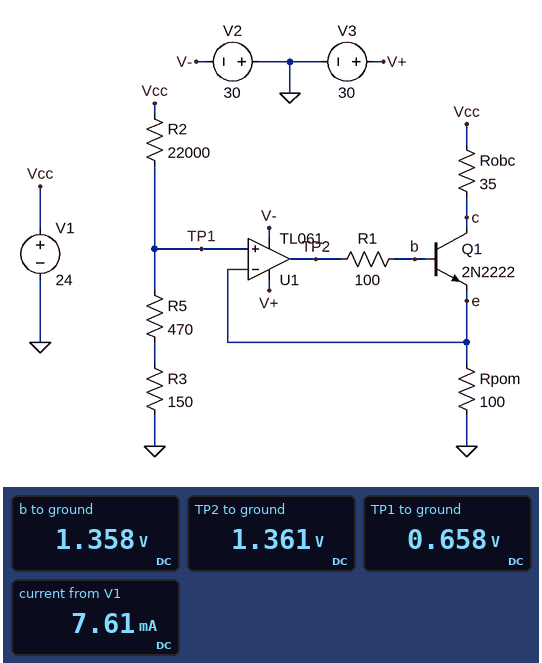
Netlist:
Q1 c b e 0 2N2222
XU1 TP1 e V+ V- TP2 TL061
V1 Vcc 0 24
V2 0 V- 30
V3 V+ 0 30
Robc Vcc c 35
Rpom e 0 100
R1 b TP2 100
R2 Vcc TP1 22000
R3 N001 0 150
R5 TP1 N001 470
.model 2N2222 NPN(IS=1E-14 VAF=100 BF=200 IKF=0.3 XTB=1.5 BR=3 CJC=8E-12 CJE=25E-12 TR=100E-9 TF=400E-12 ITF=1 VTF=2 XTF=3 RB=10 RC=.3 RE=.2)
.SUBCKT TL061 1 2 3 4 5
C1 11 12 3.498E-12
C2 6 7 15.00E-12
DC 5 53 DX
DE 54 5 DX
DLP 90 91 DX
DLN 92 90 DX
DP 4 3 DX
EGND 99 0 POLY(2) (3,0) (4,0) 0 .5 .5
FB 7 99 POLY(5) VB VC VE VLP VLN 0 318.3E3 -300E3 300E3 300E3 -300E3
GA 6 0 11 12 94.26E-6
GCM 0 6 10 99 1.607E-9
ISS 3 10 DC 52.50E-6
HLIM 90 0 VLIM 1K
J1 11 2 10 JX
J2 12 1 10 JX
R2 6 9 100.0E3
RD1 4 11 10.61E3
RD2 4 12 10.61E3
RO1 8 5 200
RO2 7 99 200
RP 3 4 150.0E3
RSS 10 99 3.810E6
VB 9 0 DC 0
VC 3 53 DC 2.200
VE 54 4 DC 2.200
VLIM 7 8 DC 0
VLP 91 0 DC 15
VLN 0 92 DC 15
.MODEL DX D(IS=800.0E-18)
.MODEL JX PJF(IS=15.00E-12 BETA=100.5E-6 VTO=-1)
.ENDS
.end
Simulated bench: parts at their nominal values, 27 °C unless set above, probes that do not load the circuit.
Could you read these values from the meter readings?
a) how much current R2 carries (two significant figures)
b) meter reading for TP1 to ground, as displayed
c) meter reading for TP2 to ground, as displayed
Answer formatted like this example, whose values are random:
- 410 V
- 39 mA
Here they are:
- 1.1 mA
- 0.658 V
- 1.361 V
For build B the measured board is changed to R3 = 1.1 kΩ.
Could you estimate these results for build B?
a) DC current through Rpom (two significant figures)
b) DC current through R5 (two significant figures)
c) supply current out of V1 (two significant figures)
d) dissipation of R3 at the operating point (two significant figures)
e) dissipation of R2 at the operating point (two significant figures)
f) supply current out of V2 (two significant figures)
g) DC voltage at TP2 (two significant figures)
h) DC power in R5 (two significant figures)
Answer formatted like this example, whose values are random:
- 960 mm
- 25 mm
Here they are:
- 16 mA
- 1.0 mA
- 17 mA
- 1.1 mW
- 23 mW
- 450 µA
- 2.3 V
- 490 µW
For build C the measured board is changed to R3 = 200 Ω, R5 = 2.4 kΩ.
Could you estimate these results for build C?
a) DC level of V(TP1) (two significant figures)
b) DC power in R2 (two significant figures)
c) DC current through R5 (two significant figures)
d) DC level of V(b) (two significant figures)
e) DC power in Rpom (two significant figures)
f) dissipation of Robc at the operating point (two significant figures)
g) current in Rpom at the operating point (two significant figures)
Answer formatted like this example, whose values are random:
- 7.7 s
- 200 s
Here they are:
- 2.5 V
- 21 mW
- 980 µA
- 3.3 V
- 64 mW
- 22 mW
- 25 mA
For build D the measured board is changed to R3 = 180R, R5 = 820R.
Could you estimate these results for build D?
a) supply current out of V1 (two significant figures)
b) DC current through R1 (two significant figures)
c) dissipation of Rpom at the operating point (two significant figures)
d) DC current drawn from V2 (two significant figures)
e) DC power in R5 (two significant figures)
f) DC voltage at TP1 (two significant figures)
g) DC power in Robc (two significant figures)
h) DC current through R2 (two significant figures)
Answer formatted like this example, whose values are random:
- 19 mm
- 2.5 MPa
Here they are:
- 11 mA
- 44 µA
- 11 mW
- 450 µA
- 890 µW
- 1.0 V
- 3.8 mW
- 1.0 mA
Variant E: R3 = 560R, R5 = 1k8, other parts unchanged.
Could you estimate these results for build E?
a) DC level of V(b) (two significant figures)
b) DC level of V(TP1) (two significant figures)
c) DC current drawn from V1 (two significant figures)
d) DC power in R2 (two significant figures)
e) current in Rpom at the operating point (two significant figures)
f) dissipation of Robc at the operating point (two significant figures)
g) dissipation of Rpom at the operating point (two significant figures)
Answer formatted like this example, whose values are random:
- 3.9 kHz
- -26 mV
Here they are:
- 3.1 V
- 2.3 V
- 24 mA
- 21 mW
- 23 mA
- 19 mW
- 54 mW
